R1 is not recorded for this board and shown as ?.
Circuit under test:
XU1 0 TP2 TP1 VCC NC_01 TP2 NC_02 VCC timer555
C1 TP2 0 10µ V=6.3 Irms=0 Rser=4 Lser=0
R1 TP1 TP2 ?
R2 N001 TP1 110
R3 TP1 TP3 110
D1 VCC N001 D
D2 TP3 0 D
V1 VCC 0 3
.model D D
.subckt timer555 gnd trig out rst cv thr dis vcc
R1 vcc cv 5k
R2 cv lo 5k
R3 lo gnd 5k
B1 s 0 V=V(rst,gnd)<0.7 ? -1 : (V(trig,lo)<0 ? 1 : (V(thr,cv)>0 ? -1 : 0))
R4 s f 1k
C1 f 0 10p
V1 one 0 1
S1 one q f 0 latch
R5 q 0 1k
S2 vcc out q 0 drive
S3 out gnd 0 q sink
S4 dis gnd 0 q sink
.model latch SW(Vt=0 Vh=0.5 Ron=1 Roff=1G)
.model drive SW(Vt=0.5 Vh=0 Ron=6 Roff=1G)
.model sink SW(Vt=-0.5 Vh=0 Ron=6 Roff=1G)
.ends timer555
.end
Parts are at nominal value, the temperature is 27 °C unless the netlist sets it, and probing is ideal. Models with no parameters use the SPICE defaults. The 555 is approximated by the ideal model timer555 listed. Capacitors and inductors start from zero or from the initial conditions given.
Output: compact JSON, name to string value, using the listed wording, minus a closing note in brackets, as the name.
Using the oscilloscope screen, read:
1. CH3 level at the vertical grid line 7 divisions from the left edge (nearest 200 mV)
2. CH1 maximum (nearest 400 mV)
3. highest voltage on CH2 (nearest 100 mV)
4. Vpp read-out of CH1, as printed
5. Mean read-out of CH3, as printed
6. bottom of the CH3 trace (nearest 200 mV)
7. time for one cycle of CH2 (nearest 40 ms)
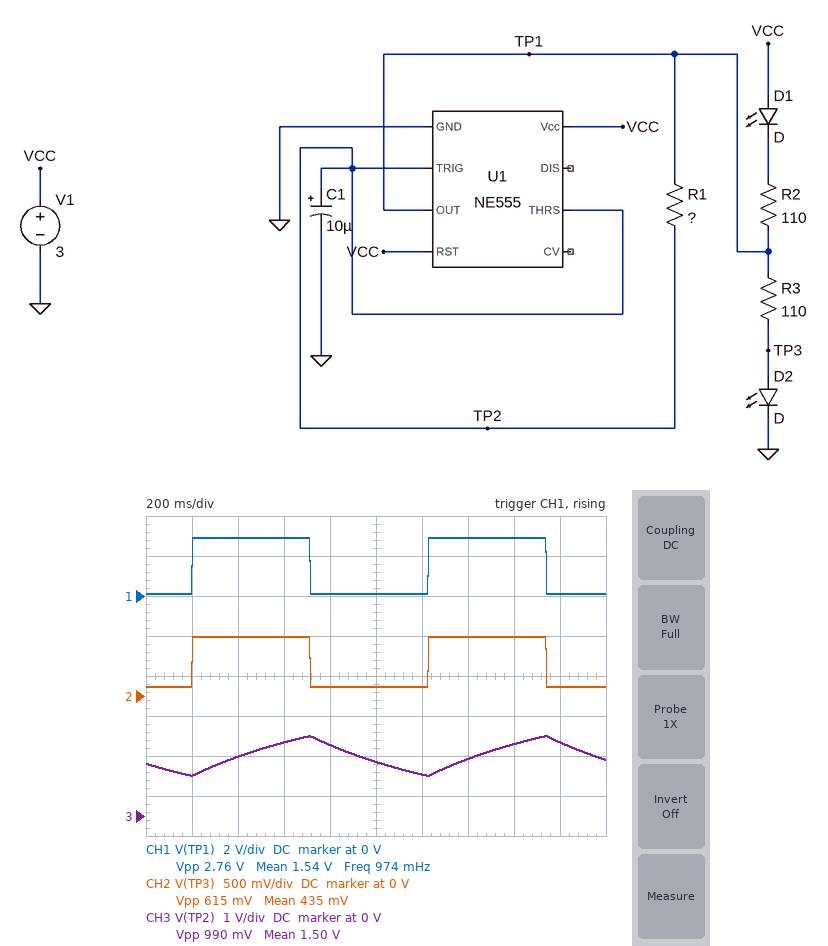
{"CH3 level at the vertical grid line 7 divisions from the left edge": "1.4 V", "CH1 maximum": "2.8 V", "highest voltage on CH2": "700 mV", "Vpp read-out of CH1, as printed": "2.76 V", "Mean read-out of CH3, as printed": "1.50 V", "bottom of the CH3 trace": "1.0 V", "time for one cycle of CH2": "1.04 s"}
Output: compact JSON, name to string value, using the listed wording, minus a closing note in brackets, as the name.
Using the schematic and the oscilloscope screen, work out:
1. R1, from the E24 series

{"R1, from the E24 series": "68 kΩ"}
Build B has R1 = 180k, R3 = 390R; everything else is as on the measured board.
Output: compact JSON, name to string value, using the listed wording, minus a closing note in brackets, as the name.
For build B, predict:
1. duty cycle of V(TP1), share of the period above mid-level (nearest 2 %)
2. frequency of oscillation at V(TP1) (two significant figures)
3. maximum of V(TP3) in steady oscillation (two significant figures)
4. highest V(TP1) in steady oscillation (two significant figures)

{"duty cycle of V(TP1), share of the period above mid-level": "48 %", "frequency of oscillation at V(TP1)": "380 mHz", "maximum of V(TP3) in steady oscillation": "700 mV", "highest V(TP1) in steady oscillation": "3.0 V"}
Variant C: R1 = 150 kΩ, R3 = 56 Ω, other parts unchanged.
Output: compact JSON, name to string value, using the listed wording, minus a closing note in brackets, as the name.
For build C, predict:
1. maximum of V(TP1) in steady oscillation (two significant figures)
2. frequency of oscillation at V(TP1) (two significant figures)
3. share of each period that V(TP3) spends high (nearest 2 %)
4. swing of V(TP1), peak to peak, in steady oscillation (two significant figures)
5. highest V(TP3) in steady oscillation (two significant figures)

{"maximum of V(TP1) in steady oscillation": "2.8 V", "frequency of oscillation at V(TP1)": "420 mHz", "share of each period that V(TP3) spends high": "52 %", "swing of V(TP1), peak to peak, in steady oscillation": "2.7 V", "highest V(TP3) in steady oscillation": "750 mV"}
